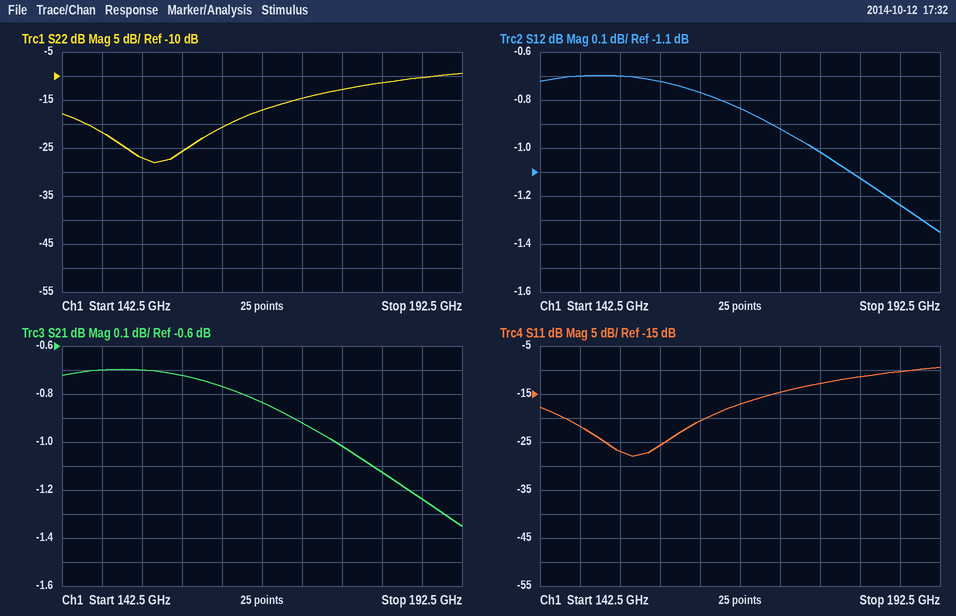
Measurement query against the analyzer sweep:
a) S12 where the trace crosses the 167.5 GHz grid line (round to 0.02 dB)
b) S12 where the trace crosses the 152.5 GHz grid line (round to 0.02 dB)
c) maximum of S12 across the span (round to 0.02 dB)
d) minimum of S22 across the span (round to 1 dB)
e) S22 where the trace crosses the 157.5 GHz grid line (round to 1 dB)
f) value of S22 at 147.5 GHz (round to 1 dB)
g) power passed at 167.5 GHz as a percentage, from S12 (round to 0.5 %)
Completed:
-0.84 dB
-0.70 dB
-0.70 dB
-28 dB
-26 dB
-22 dB
82.5 %
